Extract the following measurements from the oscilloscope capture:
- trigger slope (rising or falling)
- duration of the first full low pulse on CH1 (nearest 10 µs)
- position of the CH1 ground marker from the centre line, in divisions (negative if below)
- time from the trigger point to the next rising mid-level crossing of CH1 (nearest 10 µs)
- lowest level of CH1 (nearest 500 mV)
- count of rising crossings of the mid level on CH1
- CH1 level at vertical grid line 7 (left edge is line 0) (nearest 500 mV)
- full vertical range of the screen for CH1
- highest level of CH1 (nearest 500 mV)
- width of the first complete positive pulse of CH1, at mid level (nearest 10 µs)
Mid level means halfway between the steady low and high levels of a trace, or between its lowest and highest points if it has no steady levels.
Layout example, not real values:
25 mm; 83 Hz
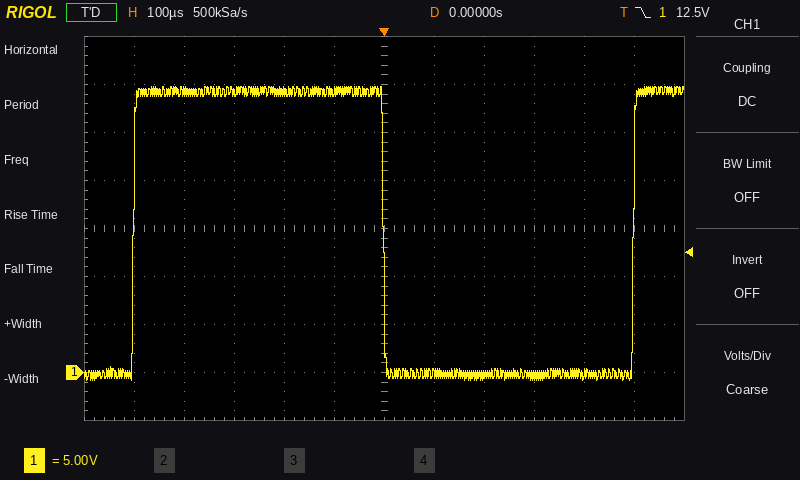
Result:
falling; 500 µs; -3.0 div; 500 µs; -1.0 V; 2; 0.0 V; 40 V; 30.0 V; 500 µs
